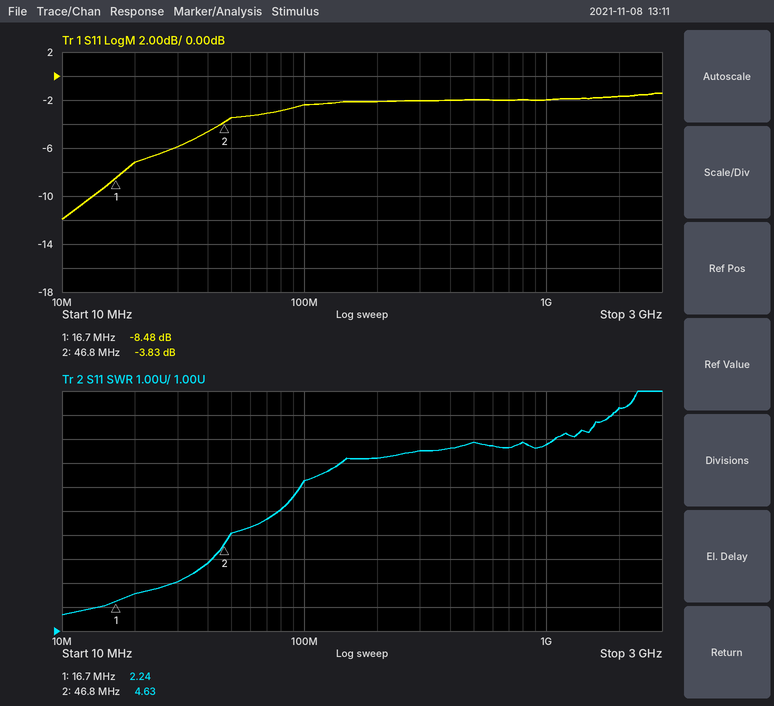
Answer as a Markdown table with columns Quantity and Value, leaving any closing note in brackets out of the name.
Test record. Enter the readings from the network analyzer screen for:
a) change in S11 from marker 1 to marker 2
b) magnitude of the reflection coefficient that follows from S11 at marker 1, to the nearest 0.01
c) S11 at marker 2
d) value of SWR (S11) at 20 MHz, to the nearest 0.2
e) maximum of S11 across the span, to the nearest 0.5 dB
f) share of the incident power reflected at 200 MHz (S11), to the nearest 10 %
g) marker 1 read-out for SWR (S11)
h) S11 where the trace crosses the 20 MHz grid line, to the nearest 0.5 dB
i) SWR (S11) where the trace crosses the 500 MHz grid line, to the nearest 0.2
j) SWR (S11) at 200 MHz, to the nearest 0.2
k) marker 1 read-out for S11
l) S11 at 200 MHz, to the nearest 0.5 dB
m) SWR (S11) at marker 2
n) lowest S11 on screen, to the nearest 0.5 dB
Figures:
| Quantity | Value |
|---|---|
| change in S11 from marker 1 to marker 2 | 4.65 dB |
| magnitude of the reflection coefficient that follows from S11 at marker 1, to the nearest 0.01 | 0.38 |
| S11 at marker 2 | -3.83 dB |
| value of SWR (S11) at 20 MHz, to the nearest 0.2 | 2.6 |
| maximum of S11 across the span, to the nearest 0.5 dB | -1.5 dB |
| share of the incident power reflected at 200 MHz (S11), to the nearest 10 % | 60 % |
| marker 1 read-out for SWR | 2.24 |
| S11 where the trace crosses the 20 MHz grid line, to the nearest 0.5 dB | -7.0 dB |
| SWR (S11) where the trace crosses the 500 MHz grid line, to the nearest 0.2 | 8.8 |
| SWR (S11) at 200 MHz, to the nearest 0.2 | 8.2 |
| marker 1 read-out for S11 | -8.48 dB |
| S11 at 200 MHz, to the nearest 0.5 dB | -2.0 dB |
| SWR (S11) at marker 2 | 4.63 |
| lowest S11 on screen, to the nearest 0.5 dB | -12.0 dB |
